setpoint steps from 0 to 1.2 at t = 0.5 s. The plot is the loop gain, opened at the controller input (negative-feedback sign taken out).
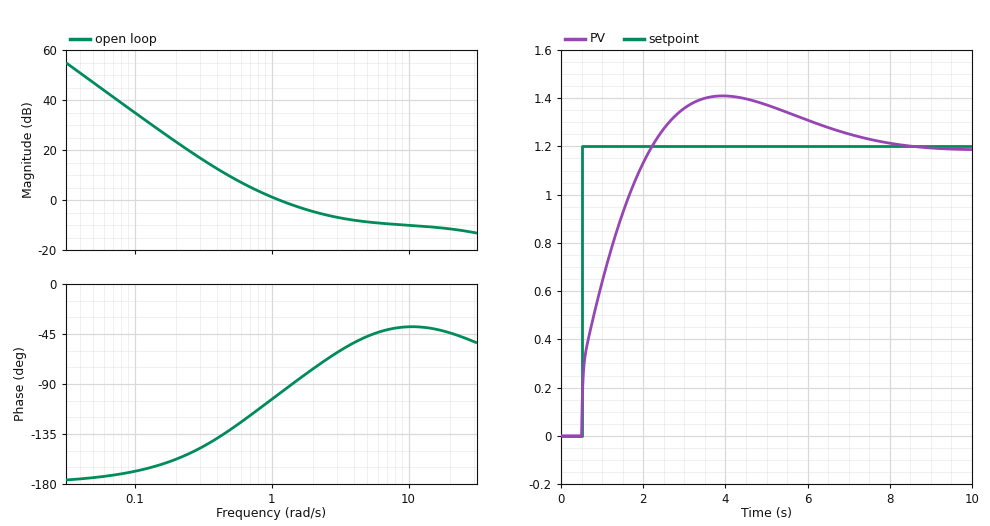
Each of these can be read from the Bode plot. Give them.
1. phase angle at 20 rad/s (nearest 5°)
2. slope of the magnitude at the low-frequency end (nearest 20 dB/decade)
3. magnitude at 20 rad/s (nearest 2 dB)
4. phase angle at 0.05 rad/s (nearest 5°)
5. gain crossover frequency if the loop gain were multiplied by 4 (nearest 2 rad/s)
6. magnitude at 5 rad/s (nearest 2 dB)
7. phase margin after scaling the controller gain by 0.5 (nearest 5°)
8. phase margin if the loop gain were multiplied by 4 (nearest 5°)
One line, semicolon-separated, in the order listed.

-45°; -40 dB/decade; -12 dB; -175°; 24 rad/s; -8 dB; 60°; 135°
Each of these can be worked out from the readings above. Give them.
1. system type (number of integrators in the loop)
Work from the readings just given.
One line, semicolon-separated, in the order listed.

2
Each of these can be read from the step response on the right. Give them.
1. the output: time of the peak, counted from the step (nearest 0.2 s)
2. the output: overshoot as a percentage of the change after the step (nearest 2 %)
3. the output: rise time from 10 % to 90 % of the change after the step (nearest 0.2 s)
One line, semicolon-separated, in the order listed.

3.4 s; 18 %; 1.4 s
